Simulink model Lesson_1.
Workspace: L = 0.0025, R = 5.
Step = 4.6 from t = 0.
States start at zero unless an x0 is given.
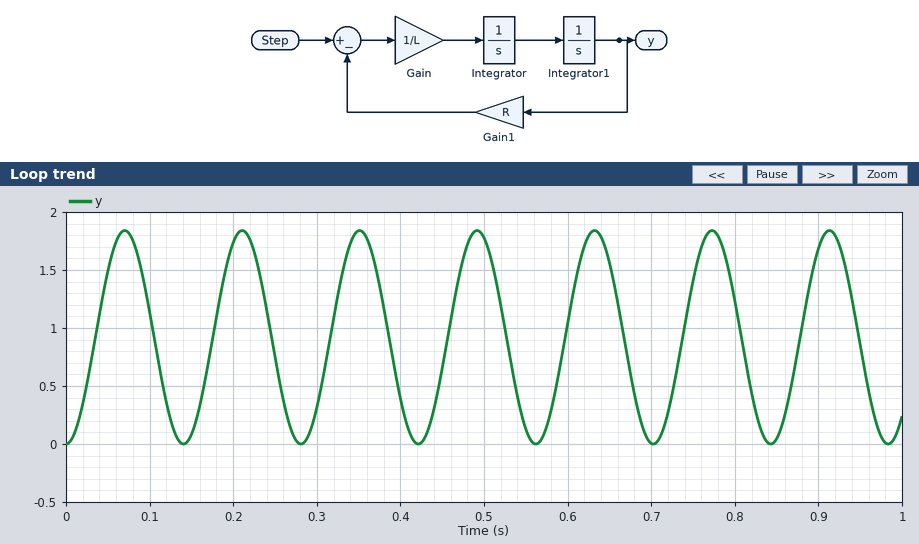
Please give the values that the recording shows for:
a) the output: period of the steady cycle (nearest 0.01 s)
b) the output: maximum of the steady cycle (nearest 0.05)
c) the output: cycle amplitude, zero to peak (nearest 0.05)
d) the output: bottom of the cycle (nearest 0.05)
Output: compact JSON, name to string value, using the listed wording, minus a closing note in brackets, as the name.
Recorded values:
{"the output: period of the steady cycle": "0.14 s", "the output: maximum of the steady cycle": "1.85", "the output: cycle amplitude, zero to peak": "0.90", "the output: bottom of the cycle": "0.00"}
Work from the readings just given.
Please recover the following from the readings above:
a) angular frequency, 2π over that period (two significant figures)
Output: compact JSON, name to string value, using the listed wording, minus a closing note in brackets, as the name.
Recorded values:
{"angular frequency, 2π over that period": "45 rad/s"}
